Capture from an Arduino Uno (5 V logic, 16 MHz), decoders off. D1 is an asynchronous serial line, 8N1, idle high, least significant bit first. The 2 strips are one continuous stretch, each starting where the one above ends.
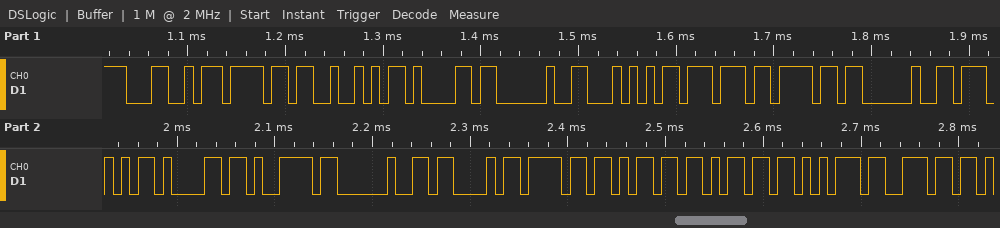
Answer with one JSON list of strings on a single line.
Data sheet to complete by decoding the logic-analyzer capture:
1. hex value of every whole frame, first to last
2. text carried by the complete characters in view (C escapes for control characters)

["4C 6F 52 61 20 54 77 6F 20 57 61 79 20 43 6F 6D 6D 75 6E", "\"LoRa Two Way Commun\""]
